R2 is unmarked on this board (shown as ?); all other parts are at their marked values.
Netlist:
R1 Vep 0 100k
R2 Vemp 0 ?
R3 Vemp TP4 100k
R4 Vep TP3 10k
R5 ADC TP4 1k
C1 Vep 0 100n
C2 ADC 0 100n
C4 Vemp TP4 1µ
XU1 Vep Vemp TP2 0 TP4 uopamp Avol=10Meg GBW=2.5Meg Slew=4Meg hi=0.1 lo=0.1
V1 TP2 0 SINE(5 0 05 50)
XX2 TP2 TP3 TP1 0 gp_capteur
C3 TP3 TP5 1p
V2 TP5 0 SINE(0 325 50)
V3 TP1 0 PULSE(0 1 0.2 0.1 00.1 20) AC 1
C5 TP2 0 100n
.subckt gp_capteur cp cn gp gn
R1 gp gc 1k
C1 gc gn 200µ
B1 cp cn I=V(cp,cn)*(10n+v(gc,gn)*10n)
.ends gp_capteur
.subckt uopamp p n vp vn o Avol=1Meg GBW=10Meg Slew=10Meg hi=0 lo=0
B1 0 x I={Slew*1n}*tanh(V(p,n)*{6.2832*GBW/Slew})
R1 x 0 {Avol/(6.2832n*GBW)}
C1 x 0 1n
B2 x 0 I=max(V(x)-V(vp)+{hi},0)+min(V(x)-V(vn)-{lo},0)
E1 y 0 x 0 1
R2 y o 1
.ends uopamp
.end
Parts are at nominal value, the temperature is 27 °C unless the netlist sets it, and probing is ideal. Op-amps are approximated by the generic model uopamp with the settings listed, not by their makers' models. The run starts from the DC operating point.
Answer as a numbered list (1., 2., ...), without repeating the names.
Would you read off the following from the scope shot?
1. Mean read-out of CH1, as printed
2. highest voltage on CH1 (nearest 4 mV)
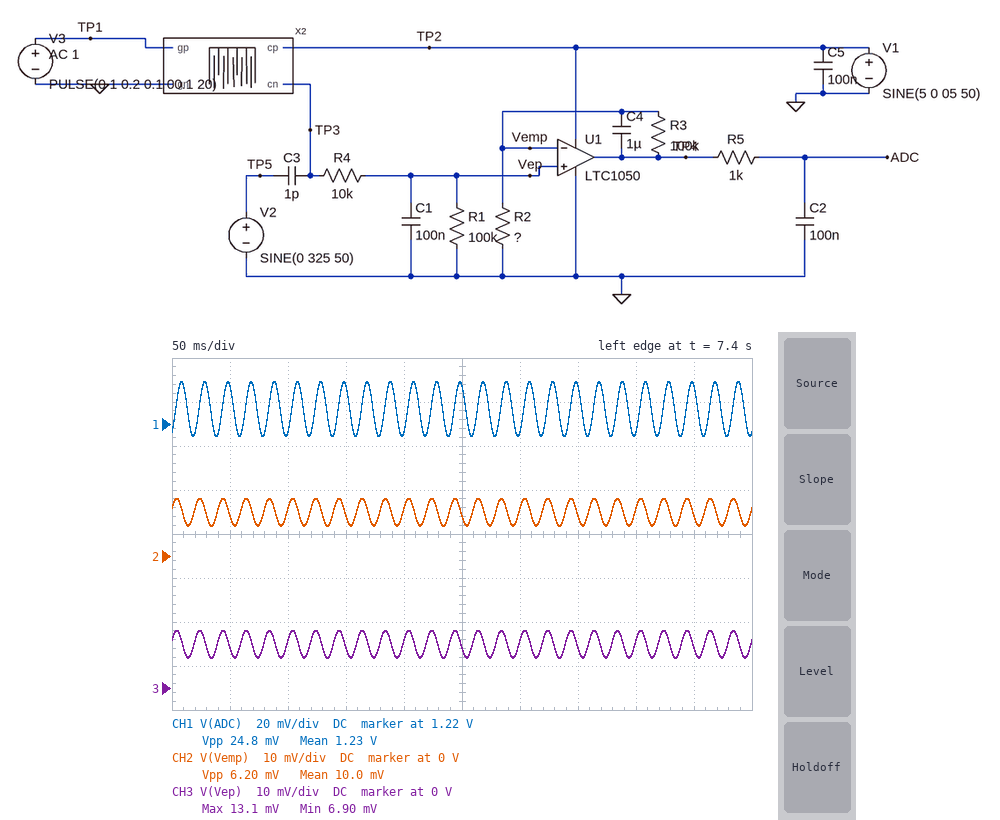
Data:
1. 1.23 V
2. 1.240 V
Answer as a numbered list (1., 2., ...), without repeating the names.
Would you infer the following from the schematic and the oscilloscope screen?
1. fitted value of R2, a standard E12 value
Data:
1. 820 Ω
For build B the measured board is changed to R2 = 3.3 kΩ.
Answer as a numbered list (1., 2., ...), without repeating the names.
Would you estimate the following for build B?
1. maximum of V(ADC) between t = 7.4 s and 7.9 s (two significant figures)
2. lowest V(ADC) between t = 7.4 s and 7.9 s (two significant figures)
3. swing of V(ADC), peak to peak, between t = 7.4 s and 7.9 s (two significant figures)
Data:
1. 320 mV
2. 310 mV
3. 8.7 mV
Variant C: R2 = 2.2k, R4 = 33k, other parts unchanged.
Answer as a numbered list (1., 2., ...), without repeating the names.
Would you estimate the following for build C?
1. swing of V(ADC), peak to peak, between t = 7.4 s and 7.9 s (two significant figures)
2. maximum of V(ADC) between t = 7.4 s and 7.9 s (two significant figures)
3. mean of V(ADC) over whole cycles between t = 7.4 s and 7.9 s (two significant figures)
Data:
1. 11 mV
2. 470 mV
3. 460 mV
